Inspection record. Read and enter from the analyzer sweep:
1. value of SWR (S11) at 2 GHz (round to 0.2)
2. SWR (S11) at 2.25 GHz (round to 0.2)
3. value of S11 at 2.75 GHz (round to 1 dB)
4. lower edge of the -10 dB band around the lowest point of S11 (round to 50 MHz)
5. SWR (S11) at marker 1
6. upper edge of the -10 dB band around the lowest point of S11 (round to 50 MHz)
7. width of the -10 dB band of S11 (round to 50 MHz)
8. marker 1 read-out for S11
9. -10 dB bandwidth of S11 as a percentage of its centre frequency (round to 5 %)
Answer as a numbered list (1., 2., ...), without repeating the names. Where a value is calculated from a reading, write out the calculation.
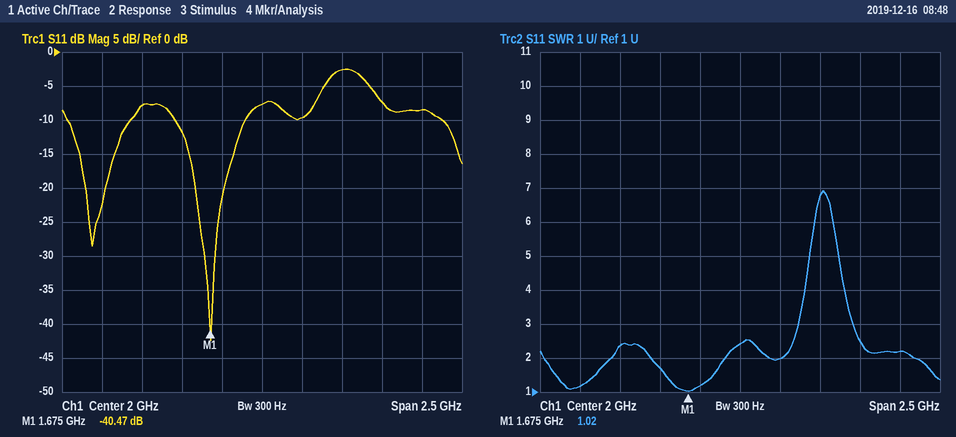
1. 2.4
2. 2.0
3. -7 dB
4. 1.45 GHz
5. 1.02
6. 1.90 GHz
7. 1.90 GHz − 1.45 GHz = 450 MHz
8. -40.47 dB
9. 450 MHz / 1.675 GHz ≈ 26.9 %, so 25 % to the nearest 5 %
